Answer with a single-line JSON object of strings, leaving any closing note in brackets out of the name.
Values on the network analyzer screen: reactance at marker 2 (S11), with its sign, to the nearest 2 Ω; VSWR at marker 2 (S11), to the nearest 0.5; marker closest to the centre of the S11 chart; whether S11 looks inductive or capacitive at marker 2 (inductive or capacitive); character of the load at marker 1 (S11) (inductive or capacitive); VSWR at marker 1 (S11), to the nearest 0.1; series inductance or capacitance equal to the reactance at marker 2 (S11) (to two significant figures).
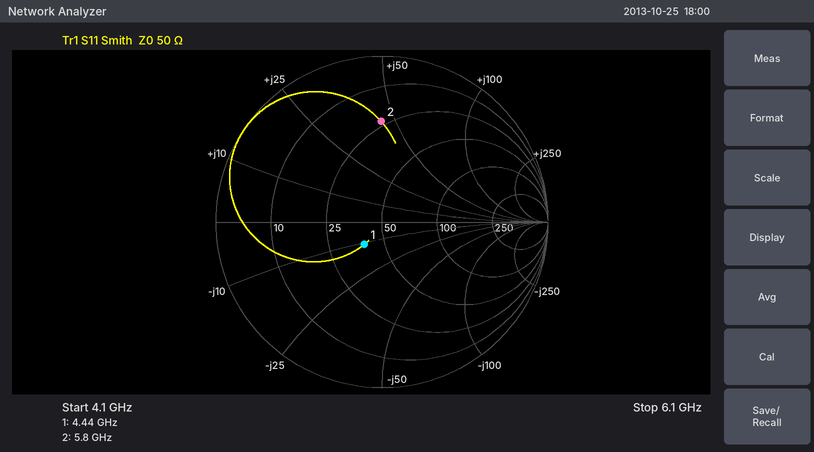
{"reactance at marker 2 (S11), with its sign, to the nearest 2 Ω": "+44 Ω", "VSWR at marker 2 (S11), to the nearest 0.5": "4.0", "marker closest to the centre of the S11 chart": "marker 1", "whether S11 looks inductive or capacitive at marker 2": "inductive", "character of the load at marker 1 (S11)": "capacitive", "VSWR at marker 1 (S11), to the nearest 0.1": "1.4", "series inductance or capacitance equal to the reactance at marker 2 (S11)": "1.2 nH"}
